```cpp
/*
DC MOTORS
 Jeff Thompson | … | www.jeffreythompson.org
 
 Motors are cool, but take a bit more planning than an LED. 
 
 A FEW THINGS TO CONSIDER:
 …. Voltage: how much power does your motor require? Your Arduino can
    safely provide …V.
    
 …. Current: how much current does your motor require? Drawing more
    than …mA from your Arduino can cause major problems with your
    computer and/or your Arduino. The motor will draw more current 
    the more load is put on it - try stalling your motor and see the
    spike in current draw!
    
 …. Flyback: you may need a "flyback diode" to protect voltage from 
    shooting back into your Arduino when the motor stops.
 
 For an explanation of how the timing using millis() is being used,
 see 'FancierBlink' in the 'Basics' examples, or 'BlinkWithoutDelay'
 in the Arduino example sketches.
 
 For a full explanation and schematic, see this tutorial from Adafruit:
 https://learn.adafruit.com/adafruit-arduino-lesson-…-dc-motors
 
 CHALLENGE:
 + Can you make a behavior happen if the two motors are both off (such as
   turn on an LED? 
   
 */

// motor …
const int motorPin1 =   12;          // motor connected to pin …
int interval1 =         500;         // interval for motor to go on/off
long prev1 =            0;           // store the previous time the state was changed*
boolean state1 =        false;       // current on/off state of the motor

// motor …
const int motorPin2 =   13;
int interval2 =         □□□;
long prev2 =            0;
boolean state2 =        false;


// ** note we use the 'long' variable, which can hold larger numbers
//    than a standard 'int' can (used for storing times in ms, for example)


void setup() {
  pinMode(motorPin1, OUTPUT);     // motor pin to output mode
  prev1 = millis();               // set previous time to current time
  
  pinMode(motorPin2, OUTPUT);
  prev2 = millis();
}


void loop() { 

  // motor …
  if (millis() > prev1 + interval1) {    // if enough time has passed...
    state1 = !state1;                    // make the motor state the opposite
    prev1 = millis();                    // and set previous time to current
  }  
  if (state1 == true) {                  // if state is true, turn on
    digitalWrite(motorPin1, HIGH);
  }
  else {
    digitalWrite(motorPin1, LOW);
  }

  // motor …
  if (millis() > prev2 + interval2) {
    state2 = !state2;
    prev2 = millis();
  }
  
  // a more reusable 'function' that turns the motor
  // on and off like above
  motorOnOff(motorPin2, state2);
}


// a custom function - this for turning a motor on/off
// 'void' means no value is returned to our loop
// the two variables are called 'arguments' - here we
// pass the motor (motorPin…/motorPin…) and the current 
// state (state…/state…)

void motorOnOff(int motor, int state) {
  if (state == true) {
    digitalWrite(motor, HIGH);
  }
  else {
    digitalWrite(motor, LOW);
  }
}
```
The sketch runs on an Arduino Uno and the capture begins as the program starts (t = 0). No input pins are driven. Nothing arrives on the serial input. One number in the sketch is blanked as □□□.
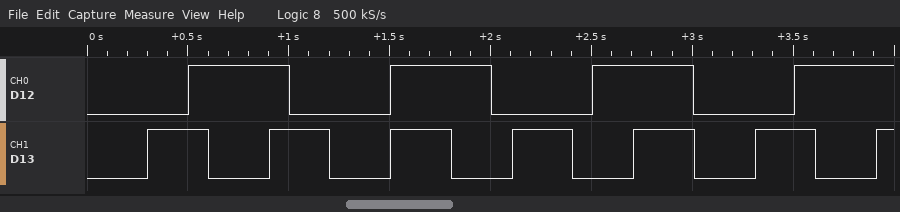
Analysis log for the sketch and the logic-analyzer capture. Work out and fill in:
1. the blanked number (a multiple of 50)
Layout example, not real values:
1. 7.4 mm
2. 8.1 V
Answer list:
1. 300
